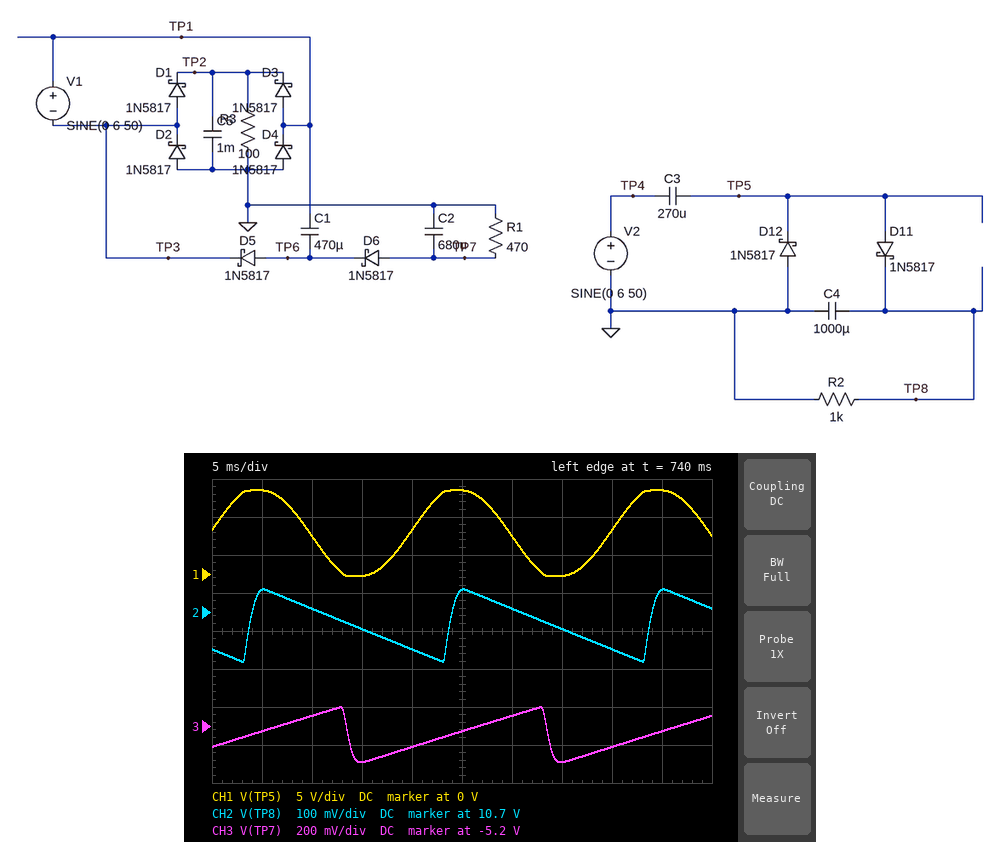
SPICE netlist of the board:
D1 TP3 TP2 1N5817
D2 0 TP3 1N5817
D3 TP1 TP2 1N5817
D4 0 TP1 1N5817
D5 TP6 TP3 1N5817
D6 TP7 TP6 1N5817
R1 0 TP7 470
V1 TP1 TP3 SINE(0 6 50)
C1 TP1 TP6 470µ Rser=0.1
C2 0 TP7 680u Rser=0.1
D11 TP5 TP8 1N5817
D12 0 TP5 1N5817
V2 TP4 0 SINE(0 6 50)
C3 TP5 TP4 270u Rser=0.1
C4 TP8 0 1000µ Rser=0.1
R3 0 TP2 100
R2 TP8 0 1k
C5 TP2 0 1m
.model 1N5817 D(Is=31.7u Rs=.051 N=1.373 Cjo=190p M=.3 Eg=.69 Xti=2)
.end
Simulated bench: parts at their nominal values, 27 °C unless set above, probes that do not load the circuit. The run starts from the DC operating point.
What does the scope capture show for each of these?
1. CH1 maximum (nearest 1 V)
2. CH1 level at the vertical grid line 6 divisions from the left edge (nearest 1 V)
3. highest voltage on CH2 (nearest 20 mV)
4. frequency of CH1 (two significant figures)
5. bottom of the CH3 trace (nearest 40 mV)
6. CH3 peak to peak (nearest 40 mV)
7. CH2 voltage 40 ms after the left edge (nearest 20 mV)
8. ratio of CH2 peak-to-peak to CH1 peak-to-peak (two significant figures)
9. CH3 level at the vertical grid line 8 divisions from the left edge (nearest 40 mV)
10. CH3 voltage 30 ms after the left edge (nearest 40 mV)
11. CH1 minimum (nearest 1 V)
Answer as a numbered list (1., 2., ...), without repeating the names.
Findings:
1. 11 V
2. 5 V
3. 10.76 V
4. 50 Hz
5. -5.40 V
6. 280 mV
7. 10.60 V
8. 0.017
9. -5.32 V
10. -5.16 V
11. 0 V
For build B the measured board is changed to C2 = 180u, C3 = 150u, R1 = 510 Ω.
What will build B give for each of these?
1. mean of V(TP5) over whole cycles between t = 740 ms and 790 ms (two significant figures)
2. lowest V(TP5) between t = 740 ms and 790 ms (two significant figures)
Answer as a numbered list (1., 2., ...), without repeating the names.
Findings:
1. 5.1 V
2. -310 mV
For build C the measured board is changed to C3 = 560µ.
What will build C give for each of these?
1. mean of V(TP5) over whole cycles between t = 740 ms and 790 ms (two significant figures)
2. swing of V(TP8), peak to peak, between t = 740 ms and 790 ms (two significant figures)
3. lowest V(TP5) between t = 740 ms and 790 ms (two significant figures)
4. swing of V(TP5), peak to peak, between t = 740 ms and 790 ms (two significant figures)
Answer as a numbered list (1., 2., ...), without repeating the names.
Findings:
1. 5.5 V
2. 200 mV
3. -330 mV
4. 12 V
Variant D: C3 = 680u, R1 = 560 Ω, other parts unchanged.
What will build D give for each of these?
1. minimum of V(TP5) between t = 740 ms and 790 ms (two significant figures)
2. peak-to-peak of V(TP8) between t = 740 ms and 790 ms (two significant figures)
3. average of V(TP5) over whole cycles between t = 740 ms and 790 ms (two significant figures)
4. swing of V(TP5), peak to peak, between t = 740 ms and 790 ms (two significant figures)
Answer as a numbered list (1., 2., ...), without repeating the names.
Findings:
1. -330 mV
2. 200 mV
3. 5.6 V
4. 12 V
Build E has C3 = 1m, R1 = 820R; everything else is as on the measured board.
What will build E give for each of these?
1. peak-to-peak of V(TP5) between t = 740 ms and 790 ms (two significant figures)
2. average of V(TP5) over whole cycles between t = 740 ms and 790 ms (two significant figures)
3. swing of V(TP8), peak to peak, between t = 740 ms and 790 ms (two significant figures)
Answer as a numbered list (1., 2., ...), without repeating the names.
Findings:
1. 12 V
2. 5.6 V
3. 200 mV
